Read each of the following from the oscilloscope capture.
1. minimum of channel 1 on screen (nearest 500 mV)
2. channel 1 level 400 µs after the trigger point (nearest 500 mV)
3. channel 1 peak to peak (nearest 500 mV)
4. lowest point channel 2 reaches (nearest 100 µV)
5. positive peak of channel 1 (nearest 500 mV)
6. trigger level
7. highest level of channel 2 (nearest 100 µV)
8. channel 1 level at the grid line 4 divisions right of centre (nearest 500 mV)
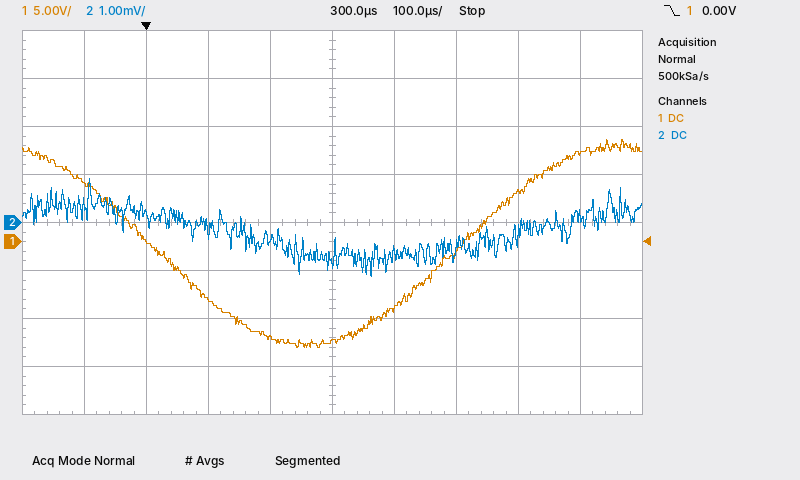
-11.0 V
-7.0 V
21.5 V
-1.1 mV
10.5 V
0.00 V
900 µV
9.0 V
